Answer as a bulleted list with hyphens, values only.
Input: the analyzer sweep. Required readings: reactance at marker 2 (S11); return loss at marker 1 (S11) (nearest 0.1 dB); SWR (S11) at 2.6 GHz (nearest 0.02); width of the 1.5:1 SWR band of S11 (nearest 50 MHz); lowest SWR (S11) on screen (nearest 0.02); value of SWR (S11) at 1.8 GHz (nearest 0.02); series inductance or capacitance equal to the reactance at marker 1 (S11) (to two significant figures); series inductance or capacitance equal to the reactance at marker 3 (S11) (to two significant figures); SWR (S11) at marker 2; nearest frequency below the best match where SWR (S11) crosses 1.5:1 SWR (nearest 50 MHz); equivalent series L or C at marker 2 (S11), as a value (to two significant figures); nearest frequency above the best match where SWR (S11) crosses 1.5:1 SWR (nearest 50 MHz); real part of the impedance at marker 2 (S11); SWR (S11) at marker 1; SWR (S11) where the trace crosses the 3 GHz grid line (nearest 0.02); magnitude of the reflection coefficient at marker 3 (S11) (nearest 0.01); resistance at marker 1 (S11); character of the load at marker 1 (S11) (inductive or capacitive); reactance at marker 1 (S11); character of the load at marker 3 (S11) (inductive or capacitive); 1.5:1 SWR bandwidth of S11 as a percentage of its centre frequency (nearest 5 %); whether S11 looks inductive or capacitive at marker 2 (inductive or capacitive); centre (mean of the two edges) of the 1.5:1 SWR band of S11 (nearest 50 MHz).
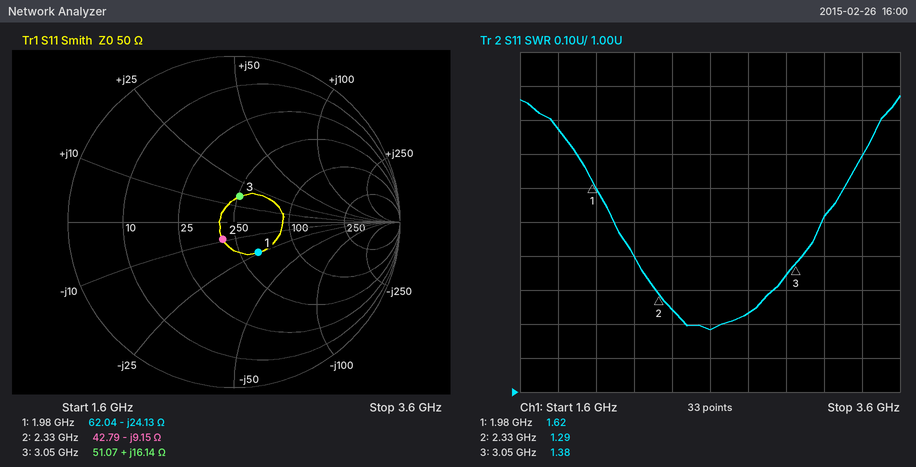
- -9.15 Ω
- 12.6 dB
- 1.18
- 1.10 GHz
- 1.18
- 1.78
- 3.3 pF
- 840 pH
- 1.29
- 2.10 GHz
- 7.5 pF
- 3.20 GHz
- 42.79 Ω
- 1.62
- 1.34
- 0.16
- 62.04 Ω
- capacitive
- -24.13 Ω
- inductive
- 40 %
- capacitive
- 2.65 GHz
